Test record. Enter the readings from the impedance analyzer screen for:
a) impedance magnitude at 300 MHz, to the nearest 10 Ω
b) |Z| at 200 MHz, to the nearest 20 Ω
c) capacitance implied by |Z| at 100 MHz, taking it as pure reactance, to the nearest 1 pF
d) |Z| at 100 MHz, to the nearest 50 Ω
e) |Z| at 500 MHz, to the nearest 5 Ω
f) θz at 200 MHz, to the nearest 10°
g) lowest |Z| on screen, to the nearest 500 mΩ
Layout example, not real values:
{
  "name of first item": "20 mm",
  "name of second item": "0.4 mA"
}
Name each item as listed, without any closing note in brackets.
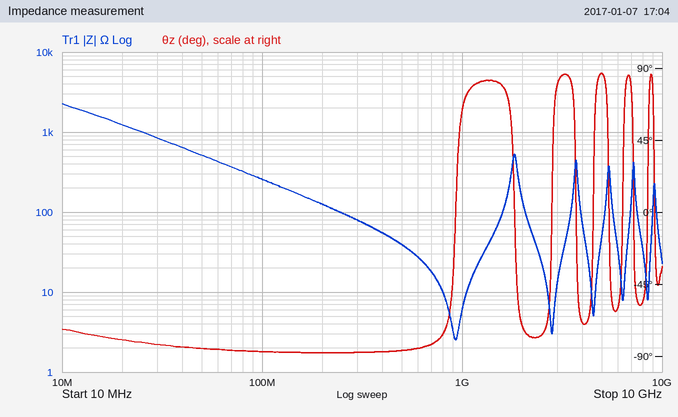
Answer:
{
  "impedance magnitude at 300 MHz, to the nearest 10 Ω": "80 Ω",
  "|Z| at 200 MHz, to the nearest 20 Ω": "120 Ω",
  "capacitance implied by |Z| at 100 MHz, taking it as pure reactance, to the nearest 1 pF": "6 pF",
  "|Z| at 100 MHz, to the nearest 50 Ω": "250 Ω",
  "|Z| at 500 MHz, to the nearest 5 Ω": "40 Ω",
  "θz at 200 MHz, to the nearest 10°": "-90°",
  "lowest |Z| on screen, to the nearest 500 mΩ": "2.5 Ω"
}
